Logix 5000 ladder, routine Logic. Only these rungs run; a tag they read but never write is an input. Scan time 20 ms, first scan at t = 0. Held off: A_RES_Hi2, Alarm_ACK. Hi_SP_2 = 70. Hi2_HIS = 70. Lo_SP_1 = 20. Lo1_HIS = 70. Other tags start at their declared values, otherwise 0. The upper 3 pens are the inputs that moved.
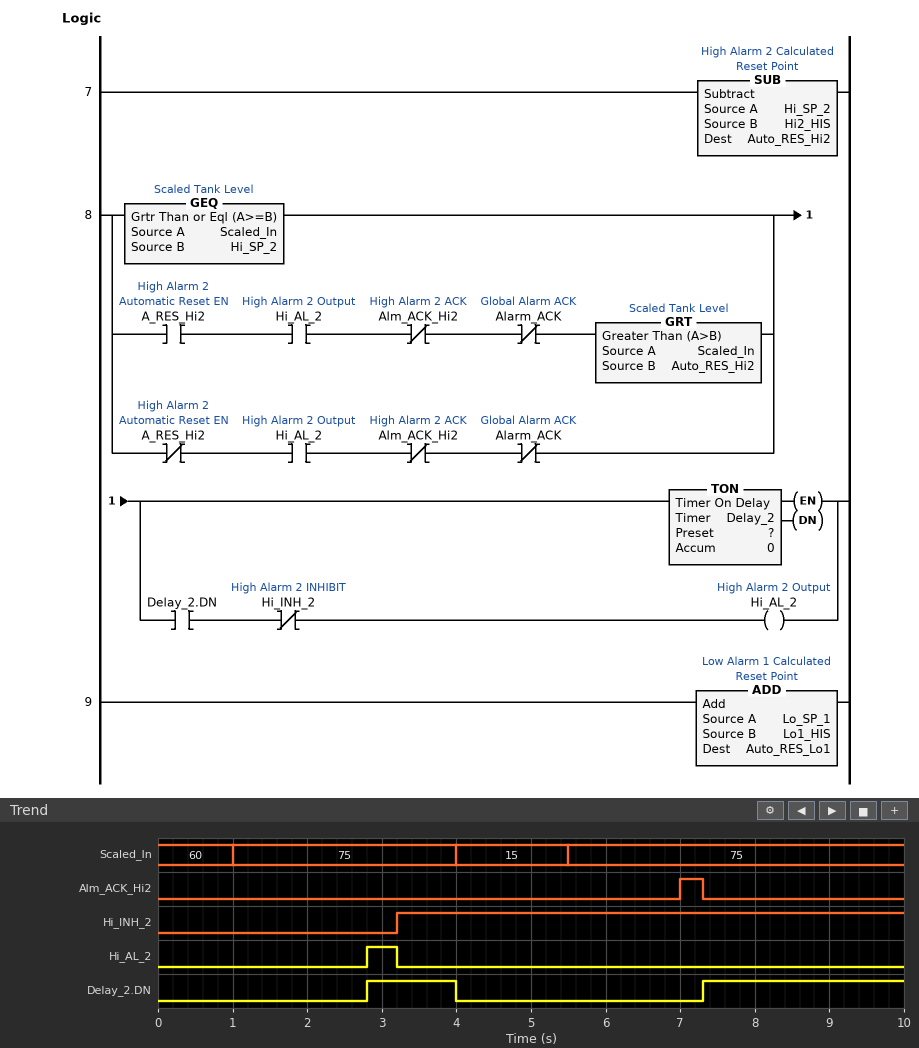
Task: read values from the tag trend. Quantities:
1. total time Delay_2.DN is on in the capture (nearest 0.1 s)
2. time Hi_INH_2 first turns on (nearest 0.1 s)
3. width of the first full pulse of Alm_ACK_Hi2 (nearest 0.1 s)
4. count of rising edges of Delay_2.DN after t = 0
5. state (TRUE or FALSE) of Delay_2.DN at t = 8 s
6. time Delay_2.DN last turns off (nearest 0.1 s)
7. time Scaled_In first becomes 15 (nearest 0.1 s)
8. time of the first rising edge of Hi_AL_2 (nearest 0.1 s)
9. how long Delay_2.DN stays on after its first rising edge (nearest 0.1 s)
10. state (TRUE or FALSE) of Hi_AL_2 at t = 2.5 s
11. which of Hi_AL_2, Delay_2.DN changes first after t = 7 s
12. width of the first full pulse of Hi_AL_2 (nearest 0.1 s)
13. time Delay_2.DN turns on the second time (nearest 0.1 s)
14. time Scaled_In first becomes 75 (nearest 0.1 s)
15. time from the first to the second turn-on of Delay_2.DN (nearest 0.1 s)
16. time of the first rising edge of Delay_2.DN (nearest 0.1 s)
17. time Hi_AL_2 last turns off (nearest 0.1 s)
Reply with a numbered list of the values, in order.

1. 3.9 s
2. 3.2 s
3. 0.3 s
4. 2
5. TRUE
6. 4.0 s
7. 4.0 s
8. 2.8 s
9. 1.2 s
10. FALSE
11. Delay_2.DN
12. 0.4 s
13. 7.3 s
14. 1.0 s
15. 4.5 s
16. 2.8 s
17. 3.2 s
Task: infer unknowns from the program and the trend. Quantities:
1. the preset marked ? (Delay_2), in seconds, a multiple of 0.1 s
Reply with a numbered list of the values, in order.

1. 1.8 s
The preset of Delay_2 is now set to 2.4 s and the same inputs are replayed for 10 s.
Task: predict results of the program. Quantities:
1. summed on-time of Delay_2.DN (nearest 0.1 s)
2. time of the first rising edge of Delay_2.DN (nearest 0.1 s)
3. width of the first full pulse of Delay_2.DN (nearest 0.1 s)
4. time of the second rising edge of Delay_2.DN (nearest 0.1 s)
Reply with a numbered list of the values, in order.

1. 2.7 s
2. 3.4 s
3. 0.6 s
4. 7.9 s
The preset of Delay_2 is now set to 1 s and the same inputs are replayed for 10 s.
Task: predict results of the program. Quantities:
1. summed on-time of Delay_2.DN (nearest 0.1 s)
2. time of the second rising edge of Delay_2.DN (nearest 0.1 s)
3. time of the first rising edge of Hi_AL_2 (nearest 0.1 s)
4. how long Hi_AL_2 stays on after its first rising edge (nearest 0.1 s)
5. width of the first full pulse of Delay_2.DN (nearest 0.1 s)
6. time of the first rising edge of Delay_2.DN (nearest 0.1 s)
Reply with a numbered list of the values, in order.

1. 5.5 s
2. 6.5 s
3. 2.0 s
4. 1.2 s
5. 2.0 s
6. 2.0 s
